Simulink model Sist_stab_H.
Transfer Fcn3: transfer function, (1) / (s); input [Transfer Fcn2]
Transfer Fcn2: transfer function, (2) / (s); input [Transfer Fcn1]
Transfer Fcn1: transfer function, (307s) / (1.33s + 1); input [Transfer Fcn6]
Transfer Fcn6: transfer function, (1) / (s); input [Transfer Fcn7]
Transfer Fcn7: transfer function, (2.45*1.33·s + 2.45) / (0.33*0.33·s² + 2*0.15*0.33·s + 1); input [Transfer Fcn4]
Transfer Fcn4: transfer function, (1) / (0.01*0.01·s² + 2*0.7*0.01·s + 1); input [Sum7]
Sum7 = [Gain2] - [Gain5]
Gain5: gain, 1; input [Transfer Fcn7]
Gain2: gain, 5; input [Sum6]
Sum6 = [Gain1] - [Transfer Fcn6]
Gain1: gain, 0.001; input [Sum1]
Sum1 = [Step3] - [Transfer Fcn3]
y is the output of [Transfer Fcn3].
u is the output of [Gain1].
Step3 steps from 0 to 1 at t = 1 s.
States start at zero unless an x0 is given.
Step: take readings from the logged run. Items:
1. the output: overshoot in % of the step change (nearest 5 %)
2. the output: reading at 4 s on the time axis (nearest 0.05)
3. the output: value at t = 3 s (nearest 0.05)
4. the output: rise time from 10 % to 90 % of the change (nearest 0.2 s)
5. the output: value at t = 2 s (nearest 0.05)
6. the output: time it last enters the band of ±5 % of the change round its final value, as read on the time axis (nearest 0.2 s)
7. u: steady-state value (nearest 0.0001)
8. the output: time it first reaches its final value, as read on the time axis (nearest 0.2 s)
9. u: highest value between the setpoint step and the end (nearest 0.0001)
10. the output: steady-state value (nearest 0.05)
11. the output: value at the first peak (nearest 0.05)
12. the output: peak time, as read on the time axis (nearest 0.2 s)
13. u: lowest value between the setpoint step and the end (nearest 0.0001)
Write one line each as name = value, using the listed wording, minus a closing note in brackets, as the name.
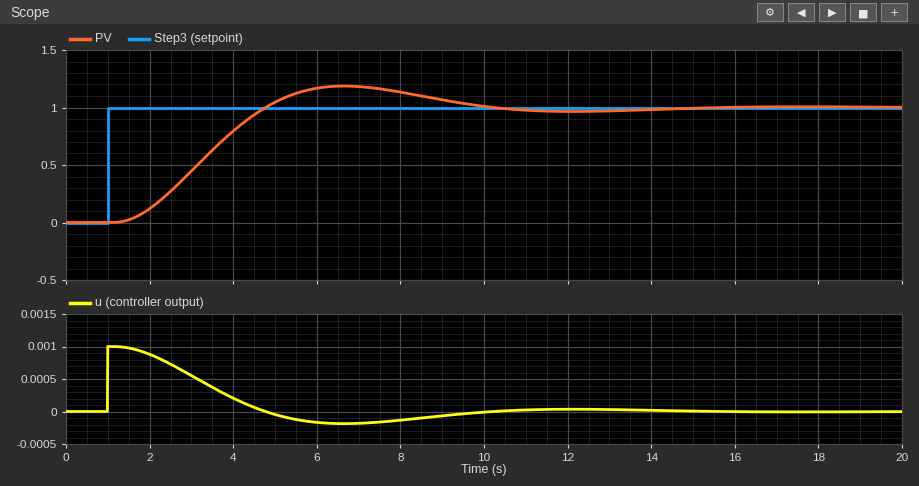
the output: overshoot in % of the step change = 20 %
the output: reading at 4 s on the time axis = 0.80
the output: value at t = 3 s = 0.45
the output: rise time from 10 % to 90 % of the change = 2.4 s
the output: value at t = 2 s = 0.10
the output: time it last enters the band of ±5 % of the change round its final value, as read on the time axis = 9.2 s
u: steady-state value = 0.0000
the output: time it first reaches its final value, as read on the time axis = 4.8 s
u: highest value between the setpoint step and the end = 0.0010
the output: steady-state value = 1.00
the output: value at the first peak = 1.20
the output: peak time, as read on the time axis = 6.6 s
u: lowest value between the setpoint step and the end = -0.0002
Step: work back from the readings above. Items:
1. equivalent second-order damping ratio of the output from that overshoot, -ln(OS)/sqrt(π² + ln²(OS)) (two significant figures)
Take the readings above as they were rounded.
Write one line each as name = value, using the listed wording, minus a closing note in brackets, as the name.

equivalent second-order damping ratio of the output from that overshoot, -ln(OS)/sqrt(π² + ln²(OS)) = 0.46
